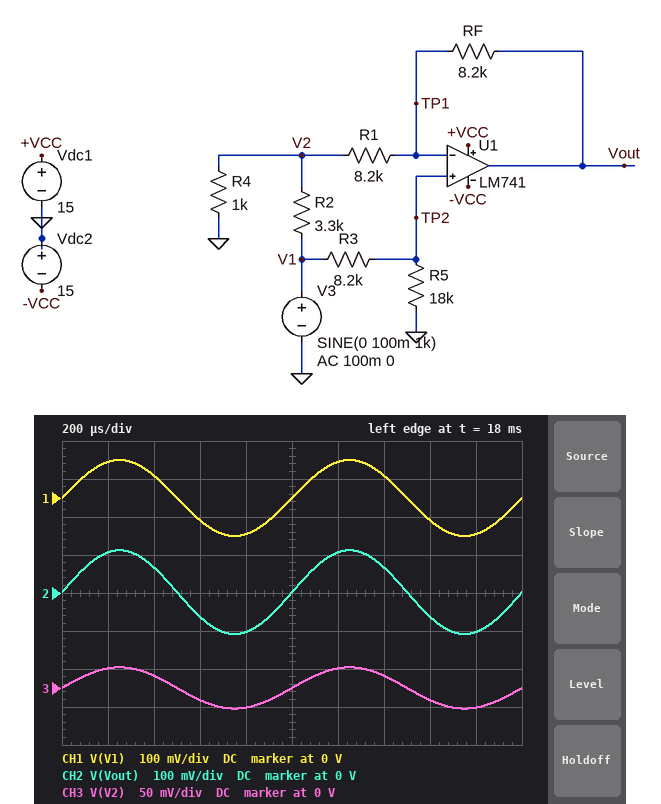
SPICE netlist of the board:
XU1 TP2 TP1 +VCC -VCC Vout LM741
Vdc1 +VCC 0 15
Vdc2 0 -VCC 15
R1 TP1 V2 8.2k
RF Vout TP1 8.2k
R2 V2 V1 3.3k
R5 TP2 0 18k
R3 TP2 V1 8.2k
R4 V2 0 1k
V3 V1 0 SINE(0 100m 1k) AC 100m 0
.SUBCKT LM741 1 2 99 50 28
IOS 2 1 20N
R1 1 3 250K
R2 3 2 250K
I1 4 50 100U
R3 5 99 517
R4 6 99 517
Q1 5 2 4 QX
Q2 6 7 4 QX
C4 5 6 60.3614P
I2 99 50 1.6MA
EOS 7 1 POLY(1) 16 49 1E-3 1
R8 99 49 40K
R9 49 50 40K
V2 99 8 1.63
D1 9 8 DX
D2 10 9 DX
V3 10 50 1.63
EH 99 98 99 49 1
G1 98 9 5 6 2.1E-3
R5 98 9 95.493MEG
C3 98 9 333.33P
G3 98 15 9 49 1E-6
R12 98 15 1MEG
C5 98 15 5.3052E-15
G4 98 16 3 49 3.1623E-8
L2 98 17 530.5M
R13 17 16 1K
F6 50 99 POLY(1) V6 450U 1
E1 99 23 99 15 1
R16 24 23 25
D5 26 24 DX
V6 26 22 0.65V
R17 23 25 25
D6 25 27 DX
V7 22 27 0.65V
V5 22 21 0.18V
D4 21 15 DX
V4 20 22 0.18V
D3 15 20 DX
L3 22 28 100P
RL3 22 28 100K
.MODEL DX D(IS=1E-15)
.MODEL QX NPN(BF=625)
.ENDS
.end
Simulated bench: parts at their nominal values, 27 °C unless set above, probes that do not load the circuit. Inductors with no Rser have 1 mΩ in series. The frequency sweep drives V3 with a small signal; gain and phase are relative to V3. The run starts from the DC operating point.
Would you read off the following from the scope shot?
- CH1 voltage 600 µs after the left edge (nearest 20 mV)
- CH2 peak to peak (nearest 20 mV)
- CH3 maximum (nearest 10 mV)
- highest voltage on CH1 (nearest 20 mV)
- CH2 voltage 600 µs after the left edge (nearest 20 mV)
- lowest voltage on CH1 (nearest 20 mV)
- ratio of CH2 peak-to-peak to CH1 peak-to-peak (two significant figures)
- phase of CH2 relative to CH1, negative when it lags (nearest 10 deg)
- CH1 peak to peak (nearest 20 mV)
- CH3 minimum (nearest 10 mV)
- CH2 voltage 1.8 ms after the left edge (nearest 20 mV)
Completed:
-60 mV
220 mV
30 mV
100 mV
-60 mV
-100 mV
1.1
0 deg
200 mV
-30 mV
-100 mV
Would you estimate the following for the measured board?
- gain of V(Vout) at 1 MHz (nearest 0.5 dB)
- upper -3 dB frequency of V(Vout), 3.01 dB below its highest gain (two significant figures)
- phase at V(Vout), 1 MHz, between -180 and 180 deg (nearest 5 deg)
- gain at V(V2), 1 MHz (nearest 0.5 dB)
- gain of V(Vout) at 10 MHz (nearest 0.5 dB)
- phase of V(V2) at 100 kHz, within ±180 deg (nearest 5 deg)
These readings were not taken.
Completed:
-5.0 dB
650 kHz
-80 deg
-13.0 dB
-37.0 dB
0 deg
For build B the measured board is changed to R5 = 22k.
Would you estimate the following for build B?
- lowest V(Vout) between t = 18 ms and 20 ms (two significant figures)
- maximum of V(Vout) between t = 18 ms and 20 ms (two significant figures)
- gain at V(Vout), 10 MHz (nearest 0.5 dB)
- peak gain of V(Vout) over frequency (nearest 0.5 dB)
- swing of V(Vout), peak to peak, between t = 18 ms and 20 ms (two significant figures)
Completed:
-120 mV
120 mV
-36.5 dB
1.5 dB
240 mV
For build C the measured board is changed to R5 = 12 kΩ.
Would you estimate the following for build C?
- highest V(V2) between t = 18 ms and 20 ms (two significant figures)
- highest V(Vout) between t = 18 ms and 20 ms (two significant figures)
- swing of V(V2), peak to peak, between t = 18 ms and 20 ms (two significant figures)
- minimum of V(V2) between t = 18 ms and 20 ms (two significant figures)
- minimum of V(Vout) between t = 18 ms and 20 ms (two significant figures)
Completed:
26 mV
95 mV
53 mV
-26 mV
-90 mV
